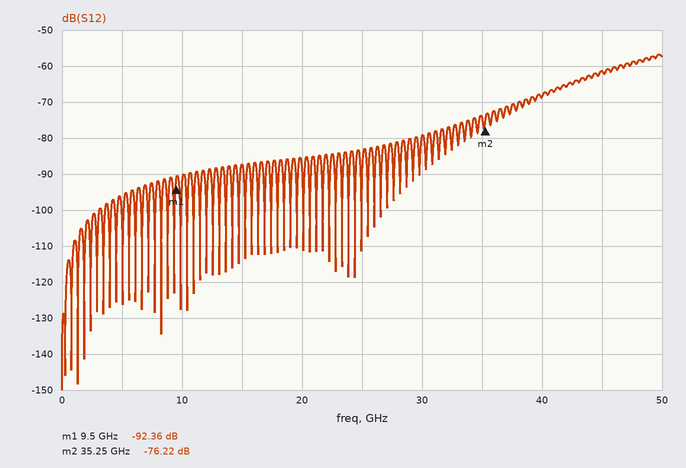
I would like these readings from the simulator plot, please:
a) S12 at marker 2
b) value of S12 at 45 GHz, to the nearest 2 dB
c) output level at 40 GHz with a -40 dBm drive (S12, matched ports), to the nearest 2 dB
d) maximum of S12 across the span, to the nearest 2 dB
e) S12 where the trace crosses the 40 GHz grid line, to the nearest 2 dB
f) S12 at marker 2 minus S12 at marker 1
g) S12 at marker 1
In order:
-76.22 dB
-62 dB
-108 dBm
-56 dB
-68 dB
16.14 dB
-92.36 dB
